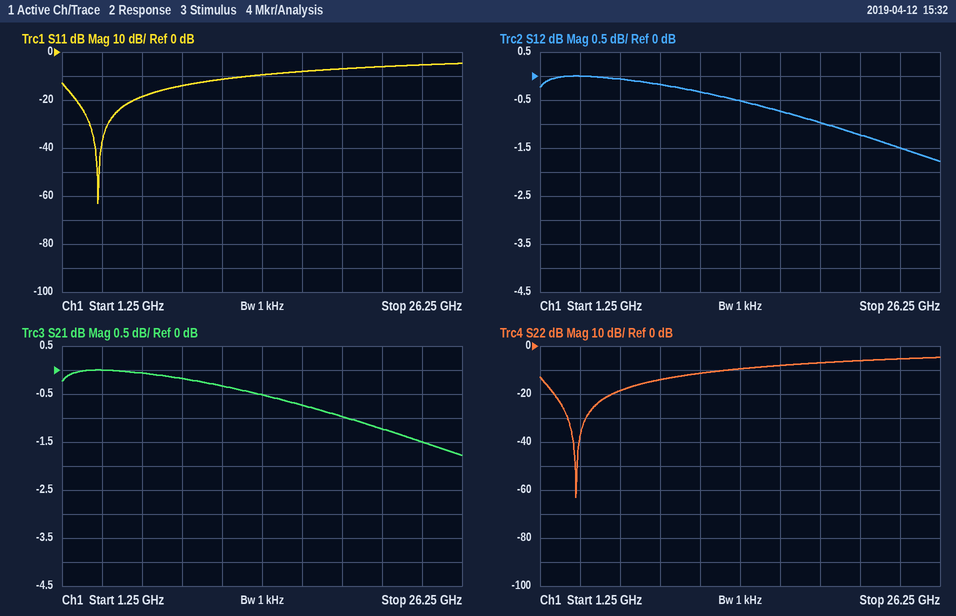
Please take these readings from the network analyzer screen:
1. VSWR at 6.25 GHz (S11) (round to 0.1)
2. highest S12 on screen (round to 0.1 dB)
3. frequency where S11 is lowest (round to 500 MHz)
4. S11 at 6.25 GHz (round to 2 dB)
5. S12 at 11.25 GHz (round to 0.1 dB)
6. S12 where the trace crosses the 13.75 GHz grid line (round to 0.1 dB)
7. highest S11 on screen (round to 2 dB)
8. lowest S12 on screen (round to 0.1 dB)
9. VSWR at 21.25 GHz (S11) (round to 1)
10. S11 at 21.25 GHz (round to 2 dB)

1.3
0.0 dB
3.5 GHz
-18 dB
-0.3 dB
-0.5 dB
-4 dB
-1.8 dB
3
-6 dB
